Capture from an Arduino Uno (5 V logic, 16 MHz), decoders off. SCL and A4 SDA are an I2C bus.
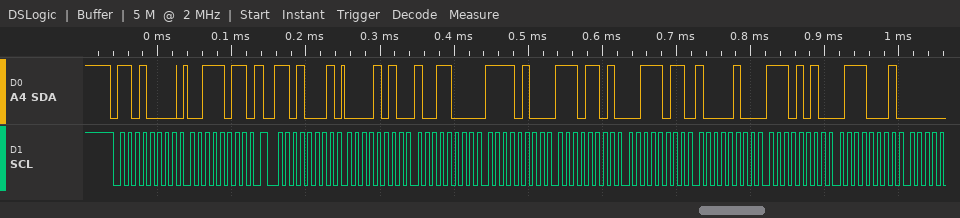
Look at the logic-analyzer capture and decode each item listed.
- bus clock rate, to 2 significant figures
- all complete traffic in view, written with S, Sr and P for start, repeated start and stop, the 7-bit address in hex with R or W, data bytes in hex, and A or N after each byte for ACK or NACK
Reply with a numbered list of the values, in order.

1. 100 kHz
2. S 68W A 3B A Sr 68R A 0A A 98 A F4 A ED A 3B A 84 A EA A 71 A
